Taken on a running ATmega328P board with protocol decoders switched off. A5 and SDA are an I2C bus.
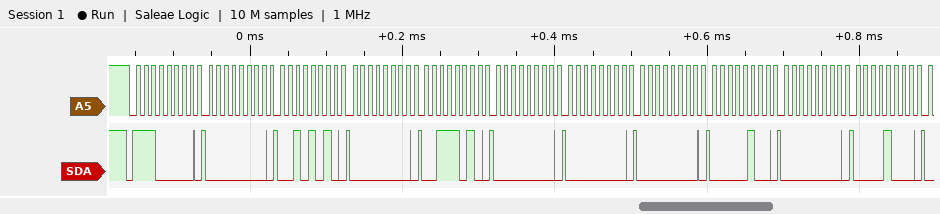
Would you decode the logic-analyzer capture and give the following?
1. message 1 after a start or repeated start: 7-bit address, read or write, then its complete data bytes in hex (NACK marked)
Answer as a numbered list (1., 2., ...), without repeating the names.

1. 0x70 write: 00 2A 00 3A 00 00 00 04 00 08
